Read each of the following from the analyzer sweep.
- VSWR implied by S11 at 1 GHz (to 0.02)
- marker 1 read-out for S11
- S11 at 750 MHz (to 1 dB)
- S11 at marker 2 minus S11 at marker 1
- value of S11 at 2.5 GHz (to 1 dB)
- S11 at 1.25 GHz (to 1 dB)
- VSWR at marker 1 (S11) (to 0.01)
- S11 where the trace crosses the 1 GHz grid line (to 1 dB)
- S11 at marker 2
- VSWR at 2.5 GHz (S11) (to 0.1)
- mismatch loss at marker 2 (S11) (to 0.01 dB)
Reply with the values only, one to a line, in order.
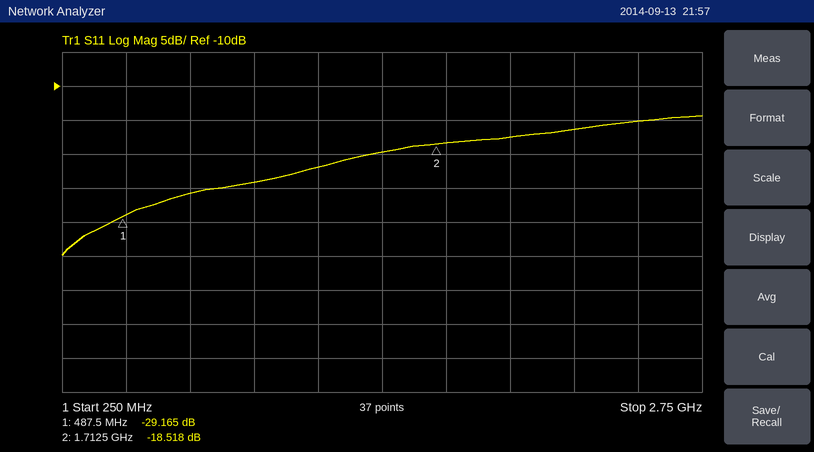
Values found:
1.14
-29.165 dB
-26 dB
10.647 dB
-15 dB
-22 dB
1.07
-24 dB
-18.518 dB
1.4
0.06 dB
